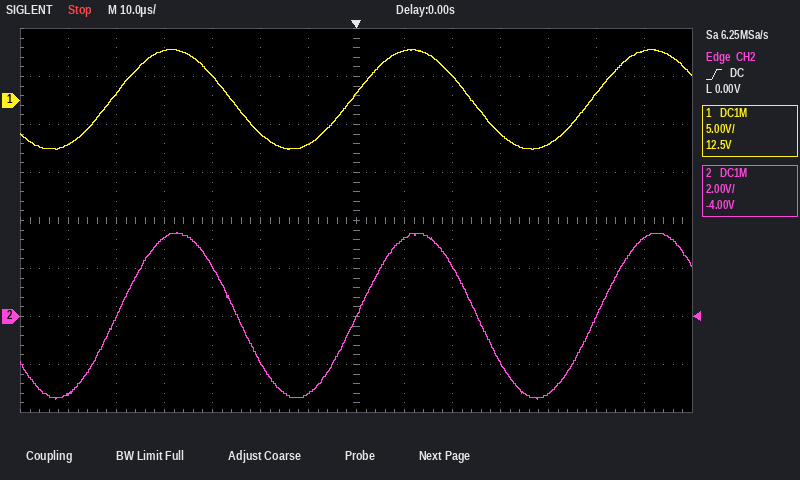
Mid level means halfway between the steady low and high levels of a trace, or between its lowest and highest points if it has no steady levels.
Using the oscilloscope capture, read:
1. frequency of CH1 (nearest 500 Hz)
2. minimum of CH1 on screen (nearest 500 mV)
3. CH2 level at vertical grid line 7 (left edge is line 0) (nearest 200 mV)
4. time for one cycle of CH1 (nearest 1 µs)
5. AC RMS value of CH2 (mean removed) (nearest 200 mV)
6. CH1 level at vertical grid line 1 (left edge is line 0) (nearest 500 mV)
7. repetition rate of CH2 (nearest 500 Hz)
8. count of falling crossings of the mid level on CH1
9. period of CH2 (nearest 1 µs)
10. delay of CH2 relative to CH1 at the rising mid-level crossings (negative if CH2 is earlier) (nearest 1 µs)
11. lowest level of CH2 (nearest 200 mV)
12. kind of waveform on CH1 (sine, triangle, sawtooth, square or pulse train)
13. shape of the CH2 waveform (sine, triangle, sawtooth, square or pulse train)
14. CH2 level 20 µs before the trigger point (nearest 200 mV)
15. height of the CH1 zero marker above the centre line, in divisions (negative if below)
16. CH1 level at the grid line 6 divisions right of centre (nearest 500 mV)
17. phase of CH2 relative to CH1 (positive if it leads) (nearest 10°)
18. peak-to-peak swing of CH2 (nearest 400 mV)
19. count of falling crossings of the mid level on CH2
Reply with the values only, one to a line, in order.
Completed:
20.0 kHz
-5.0 V
0.0 V
50 µs
2.4 V
-4.5 V
20.0 kHz
2
50 µs
+1 µs
-3.4 V
sine
sine
-1.8 V
+2.5 div
5.0 V
-10°
6.8 V
2
